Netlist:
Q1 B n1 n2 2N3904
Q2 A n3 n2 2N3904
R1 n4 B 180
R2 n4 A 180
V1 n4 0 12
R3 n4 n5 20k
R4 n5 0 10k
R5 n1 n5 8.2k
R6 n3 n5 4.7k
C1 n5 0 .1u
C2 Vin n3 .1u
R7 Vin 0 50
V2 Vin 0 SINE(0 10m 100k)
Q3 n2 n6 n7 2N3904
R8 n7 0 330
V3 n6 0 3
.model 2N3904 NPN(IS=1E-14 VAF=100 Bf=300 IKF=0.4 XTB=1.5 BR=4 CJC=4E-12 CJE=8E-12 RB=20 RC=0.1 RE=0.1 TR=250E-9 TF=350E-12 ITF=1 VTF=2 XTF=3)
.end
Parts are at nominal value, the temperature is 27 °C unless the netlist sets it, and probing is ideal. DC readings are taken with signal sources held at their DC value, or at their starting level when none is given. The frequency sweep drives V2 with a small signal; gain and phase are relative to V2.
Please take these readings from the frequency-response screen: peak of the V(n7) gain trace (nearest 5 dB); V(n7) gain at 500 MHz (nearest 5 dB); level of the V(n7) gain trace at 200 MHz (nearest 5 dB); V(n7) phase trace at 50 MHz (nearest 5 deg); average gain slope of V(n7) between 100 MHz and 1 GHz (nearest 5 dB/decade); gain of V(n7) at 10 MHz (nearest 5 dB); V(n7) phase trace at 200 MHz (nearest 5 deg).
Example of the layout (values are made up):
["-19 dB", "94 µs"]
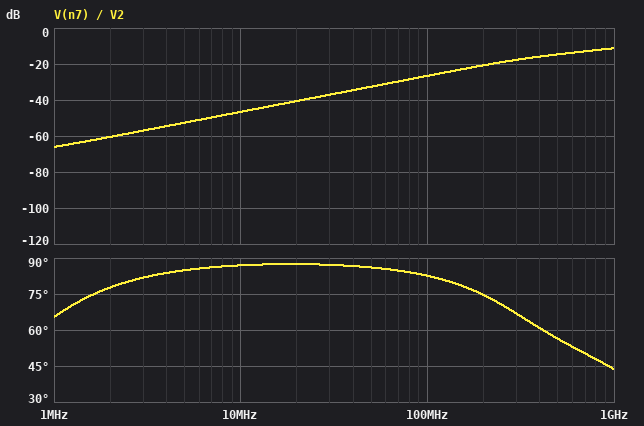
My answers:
["-10 dB", "-15 dB", "-20 dB", "85 deg", "15 dB/decade", "-45 dB", "75 deg"]
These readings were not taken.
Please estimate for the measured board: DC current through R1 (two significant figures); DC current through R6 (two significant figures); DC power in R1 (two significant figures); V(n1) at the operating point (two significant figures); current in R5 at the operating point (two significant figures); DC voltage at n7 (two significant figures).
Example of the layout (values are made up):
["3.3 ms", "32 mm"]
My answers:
["2.8 mA", "13 µA", "1.4 mW", "3.8 V", "8.7 µA", "2.3 V"]
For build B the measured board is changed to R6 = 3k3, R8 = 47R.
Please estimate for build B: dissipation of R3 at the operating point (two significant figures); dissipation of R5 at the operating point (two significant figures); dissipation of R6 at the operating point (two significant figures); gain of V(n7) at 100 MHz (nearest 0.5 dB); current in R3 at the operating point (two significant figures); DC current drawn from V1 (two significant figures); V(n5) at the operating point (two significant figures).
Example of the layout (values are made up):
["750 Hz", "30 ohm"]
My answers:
["3.9 mW", "12 µW", "25 µW", "-3.5 dB", "440 µA", "38 mA", "3.2 V"]
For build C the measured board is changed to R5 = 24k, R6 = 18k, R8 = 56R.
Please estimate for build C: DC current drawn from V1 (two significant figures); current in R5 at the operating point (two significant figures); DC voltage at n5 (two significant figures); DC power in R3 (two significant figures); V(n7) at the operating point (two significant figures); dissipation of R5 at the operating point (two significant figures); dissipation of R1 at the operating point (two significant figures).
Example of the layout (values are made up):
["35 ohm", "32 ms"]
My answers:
["24 mA", "32 µA", "3.5 V", "3.6 mW", "2.0 V", "25 µW", "19 mW"]
